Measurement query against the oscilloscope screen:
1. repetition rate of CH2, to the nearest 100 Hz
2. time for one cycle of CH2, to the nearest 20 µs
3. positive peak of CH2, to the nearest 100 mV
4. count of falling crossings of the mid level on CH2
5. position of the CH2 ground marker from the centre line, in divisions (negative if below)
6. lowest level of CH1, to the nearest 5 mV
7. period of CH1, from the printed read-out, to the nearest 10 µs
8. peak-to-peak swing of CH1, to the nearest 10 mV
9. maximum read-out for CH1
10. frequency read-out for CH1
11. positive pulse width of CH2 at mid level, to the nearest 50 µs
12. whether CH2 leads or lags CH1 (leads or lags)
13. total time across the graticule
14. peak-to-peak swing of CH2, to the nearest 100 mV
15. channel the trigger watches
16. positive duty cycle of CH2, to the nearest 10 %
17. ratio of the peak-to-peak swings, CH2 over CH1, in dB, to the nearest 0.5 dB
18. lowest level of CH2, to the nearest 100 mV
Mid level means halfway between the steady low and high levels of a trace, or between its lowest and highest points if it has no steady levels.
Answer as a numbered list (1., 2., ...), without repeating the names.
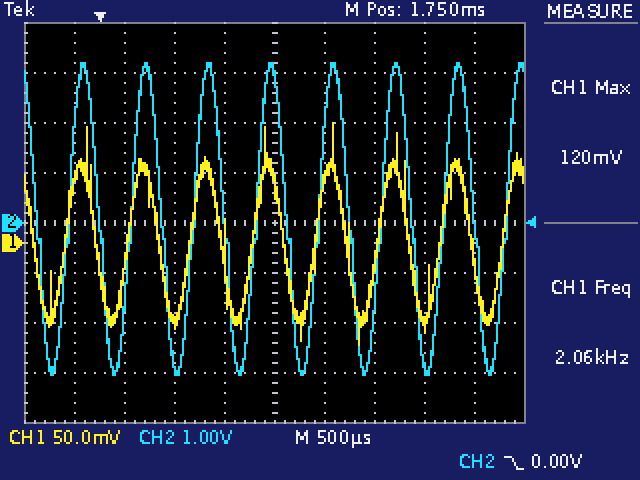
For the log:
1. 1.6 kHz
2. 620 µs
3. 3.2 V
4. 8
5. 0.0 div
6. -100 mV
7. 490 µs
8. 220 mV
9. 120 mV
10. 2.06 kHz
11. 300 µs
12. lags
13. 5 ms
14. 6.2 V
15. CH2
16. 50 %
17. 29.0 dB
18. -3.0 V
